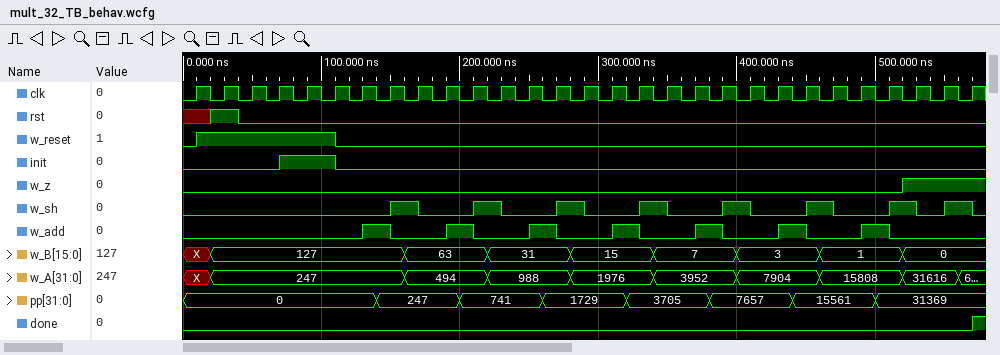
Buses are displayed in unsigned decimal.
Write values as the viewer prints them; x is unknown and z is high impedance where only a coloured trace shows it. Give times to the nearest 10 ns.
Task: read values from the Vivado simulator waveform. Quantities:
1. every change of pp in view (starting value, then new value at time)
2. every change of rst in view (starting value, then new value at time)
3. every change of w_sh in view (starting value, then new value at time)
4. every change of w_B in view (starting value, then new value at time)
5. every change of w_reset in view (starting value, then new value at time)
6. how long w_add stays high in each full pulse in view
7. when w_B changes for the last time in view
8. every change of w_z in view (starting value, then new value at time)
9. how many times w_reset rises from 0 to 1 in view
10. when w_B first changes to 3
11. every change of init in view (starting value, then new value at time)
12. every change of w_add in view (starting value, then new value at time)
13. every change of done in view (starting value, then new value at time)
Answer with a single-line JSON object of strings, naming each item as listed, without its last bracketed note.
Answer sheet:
{"every change of pp in view": "0, 247 at 140 ns, 741 at 200 ns, 1729 at 260 ns, 3705 at 320 ns, 7657 at 380 ns, 15561 at 440 ns, 31369 at 500 ns", "every change of rst in view": "x, 1 at 20 ns, 0 at 40 ns", "every change of w_sh in view": "0, 1 at 150 ns, 0 at 170 ns, 1 at 210 ns, 0 at 230 ns, 1 at 270 ns, 0 at 290 ns, 1 at 330 ns, 0 at 350 ns, 1 at 390 ns, 0 at 410 ns, 1 at 450 ns, 0 at 470 ns, 1 at 510 ns, 0 at 530 ns, 1 at 550 ns, 0 at 570 ns", "every change of w_B in view": "X, 127 at 20 ns, 63 at 160 ns, 31 at 220 ns, 15 at 280 ns, 7 at 340 ns, 3 at 400 ns, 1 at 460 ns, 0 at 520 ns", "every change of w_reset in view": "0, 1 at 10 ns, 0 at 110 ns", "how long w_add stays high in each full pulse in view": "20 ns, 20 ns, 20 ns, 20 ns, 20 ns, 20 ns, 20 ns", "when w_B changes for the last time in view": "520 ns", "every change of w_z in view": "0, 1 at 520 ns", "how many times w_reset rises from 0 to 1 in view": "1", "when w_B first changes to 3": "400 ns", "every change of init in view": "0, 1 at 70 ns, 0 at 110 ns", "every change of w_add in view": "0, 1 at 130 ns, 0 at 150 ns, 1 at 190 ns, 0 at 210 ns, 1 at 250 ns, 0 at 270 ns, 1 at 310 ns, 0 at 330 ns, 1 at 370 ns, 0 at 390 ns, 1 at 430 ns, 0 at 450 ns, 1 at 490 ns, 0 at 510 ns", "every change of done in view": "0, 1 at 570 ns"}
